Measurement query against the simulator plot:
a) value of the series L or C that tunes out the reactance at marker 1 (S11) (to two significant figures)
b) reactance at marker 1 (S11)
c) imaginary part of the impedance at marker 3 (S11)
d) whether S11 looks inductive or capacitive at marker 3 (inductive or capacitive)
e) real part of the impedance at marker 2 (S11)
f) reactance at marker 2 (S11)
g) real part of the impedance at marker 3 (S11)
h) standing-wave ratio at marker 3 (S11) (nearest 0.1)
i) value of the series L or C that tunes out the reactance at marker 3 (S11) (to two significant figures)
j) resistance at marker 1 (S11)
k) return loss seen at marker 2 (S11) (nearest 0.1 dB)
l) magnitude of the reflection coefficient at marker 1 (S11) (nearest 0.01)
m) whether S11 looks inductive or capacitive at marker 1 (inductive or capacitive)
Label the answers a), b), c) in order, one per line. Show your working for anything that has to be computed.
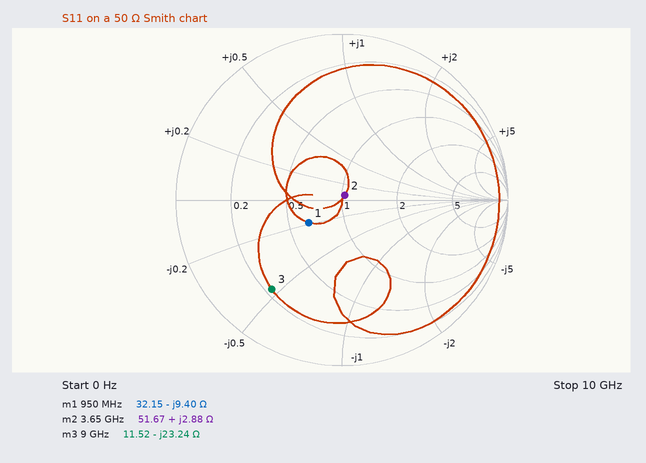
a) L = 9.4 Ω/(2π × 950 MHz) ≈ 1.6 nH
b) -9.40 Ω
c) -23.24 Ω
d) capacitive
e) 51.67 Ω
f) +2.88 Ω
g) 11.52 Ω
h) 5.3
i) L = 23.24 Ω/(2π × 9 GHz) ≈ 411 pH, so 410 pH to two significant figures
j) 32.15 Ω
k) 29.7 dB
l) 0.24
m) capacitive
